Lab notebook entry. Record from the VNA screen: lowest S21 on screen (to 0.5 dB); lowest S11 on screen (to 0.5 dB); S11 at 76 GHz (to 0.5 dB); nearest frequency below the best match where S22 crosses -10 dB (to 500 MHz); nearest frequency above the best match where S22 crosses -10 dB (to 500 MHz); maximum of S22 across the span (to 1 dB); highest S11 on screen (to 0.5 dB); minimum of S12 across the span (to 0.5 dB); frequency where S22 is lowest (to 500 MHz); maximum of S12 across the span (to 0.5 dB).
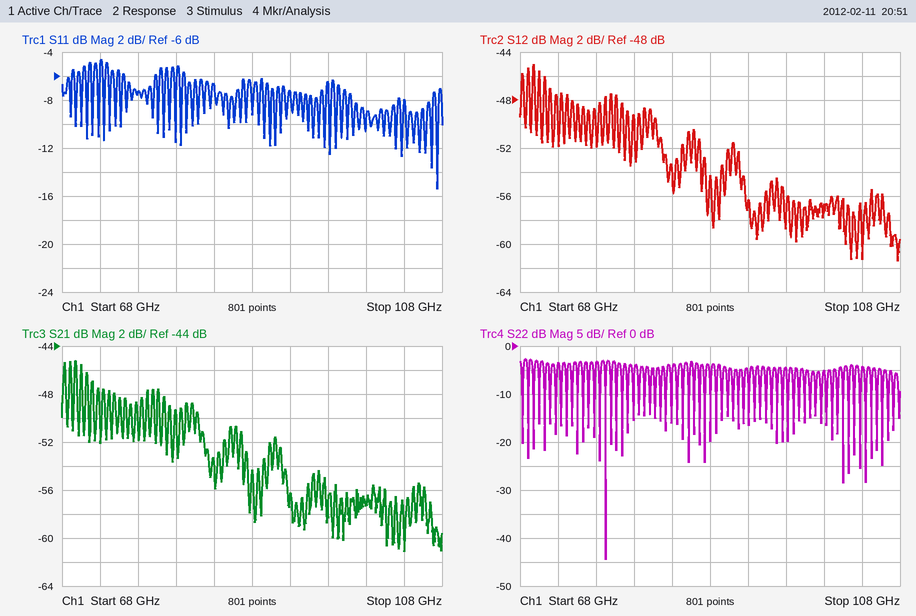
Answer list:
-61.0 dB
-15.5 dB
-7.5 dB
77.0 GHz
77.0 GHz
-3 dB
-4.5 dB
-61.5 dB
77.0 GHz
-45.0 dB
